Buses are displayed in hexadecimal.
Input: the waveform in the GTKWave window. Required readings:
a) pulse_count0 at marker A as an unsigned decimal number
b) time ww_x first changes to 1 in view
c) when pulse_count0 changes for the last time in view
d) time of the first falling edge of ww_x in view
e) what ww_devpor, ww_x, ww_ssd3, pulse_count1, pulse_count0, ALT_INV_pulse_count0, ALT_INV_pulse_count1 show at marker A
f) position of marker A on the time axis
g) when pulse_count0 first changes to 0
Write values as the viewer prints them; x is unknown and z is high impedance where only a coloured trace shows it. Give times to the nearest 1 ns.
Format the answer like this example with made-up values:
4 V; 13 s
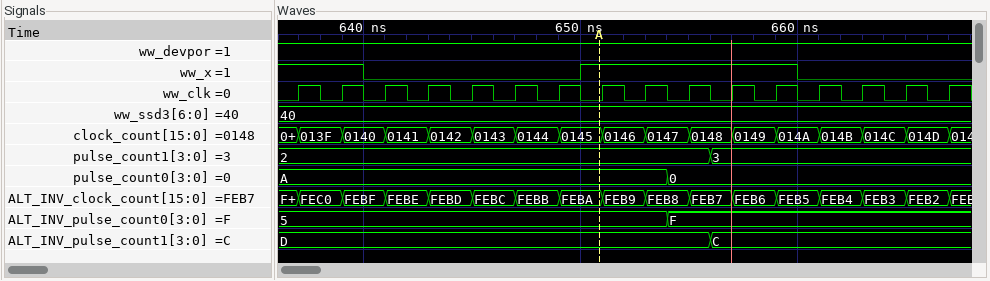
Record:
10; 650 ns; 654 ns; 640 ns; ww_devpor=1, ww_x=1, ww_ssd3=40, pulse_count1=2, pulse_count0=A, ALT_INV_pulse_count0=5, ALT_INV_pulse_count1=D; 651 ns; 654 ns
